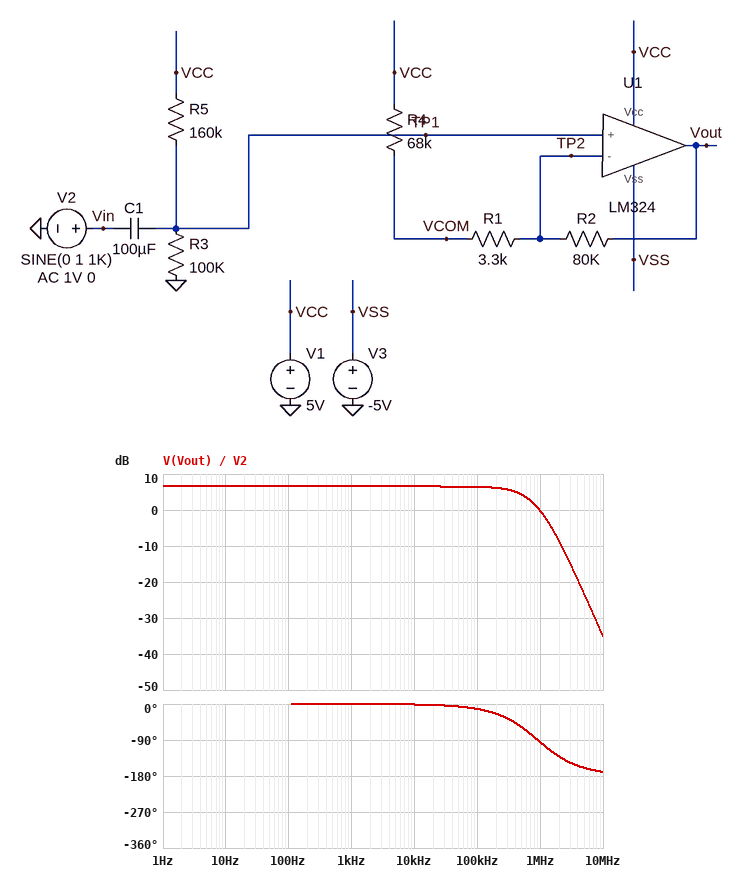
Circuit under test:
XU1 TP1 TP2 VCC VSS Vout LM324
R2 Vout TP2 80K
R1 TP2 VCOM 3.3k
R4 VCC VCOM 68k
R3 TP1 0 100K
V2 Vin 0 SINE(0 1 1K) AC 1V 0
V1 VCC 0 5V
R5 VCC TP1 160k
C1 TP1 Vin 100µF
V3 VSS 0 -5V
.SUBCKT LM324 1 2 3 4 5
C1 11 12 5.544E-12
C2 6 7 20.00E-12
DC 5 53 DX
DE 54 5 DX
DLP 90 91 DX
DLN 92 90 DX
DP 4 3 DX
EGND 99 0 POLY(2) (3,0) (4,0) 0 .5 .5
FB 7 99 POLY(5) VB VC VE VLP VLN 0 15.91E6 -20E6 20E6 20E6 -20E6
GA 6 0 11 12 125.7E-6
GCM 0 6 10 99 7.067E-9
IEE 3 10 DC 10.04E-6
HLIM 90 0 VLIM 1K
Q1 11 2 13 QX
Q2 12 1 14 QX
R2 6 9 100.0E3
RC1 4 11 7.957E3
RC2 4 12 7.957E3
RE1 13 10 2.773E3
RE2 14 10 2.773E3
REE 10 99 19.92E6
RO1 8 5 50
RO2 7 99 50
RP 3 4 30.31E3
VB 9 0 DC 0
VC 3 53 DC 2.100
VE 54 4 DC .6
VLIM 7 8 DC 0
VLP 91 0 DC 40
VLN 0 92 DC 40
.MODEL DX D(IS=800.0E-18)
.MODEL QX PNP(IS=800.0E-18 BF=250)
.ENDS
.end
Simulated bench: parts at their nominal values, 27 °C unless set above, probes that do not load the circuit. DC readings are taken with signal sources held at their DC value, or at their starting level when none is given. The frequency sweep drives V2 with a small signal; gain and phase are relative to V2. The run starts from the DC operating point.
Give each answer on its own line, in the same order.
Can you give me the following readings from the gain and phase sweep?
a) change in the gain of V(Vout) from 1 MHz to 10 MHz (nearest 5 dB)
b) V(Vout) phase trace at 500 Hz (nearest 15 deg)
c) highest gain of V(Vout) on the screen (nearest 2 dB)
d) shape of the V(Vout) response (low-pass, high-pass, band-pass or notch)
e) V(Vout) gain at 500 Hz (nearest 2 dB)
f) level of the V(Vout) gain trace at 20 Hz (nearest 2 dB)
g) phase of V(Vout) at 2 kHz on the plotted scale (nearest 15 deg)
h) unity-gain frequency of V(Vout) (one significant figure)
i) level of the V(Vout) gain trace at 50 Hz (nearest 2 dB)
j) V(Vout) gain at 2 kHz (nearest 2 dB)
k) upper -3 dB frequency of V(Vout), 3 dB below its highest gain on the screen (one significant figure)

-35 dB
0 deg
6 dB
low-pass
6 dB
6 dB
0 deg
1 MHz
6 dB
6 dB
600 kHz
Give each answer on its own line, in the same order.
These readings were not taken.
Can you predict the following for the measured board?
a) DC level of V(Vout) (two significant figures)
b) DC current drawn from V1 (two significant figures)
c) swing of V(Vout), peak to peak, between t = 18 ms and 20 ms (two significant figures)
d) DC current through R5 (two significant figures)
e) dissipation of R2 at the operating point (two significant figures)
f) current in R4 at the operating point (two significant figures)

-1.5 V
400 µA
4.2 V
19 µA
150 µW
43 µA
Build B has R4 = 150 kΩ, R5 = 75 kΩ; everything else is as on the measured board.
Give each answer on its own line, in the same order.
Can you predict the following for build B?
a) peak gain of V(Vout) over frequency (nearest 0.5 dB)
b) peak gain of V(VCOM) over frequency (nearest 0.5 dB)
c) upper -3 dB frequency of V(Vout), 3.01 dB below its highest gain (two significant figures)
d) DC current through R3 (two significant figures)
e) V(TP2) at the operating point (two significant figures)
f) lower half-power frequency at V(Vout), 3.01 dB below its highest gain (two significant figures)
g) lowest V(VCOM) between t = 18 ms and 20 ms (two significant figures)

3.5 dB
0 dB
880 kHz
29 µA
2.9 V
37 mHz
1.9 V
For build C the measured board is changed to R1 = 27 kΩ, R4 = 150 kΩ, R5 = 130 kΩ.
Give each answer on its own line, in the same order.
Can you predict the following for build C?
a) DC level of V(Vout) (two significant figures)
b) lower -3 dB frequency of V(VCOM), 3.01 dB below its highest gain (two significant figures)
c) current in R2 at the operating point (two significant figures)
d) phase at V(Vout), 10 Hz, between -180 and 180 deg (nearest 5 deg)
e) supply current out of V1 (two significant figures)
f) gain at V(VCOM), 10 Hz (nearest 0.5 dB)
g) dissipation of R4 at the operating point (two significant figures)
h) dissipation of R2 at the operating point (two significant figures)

900 mV
28 mHz
16 µA
0 deg
380 µA
-1.5 dB
38 µW
20 µW
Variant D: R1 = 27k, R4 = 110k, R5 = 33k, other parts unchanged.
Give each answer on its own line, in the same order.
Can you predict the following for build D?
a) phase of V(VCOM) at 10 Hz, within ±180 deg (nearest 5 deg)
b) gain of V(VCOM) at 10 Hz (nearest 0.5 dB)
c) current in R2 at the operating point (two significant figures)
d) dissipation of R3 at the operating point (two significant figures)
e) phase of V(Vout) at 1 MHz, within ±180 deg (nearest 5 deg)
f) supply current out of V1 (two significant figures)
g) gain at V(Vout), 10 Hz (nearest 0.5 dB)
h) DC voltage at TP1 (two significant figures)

0 deg
-2.0 dB
9.1 µA
140 µW
-85 deg
390 µA
4.0 dB
3.8 V
